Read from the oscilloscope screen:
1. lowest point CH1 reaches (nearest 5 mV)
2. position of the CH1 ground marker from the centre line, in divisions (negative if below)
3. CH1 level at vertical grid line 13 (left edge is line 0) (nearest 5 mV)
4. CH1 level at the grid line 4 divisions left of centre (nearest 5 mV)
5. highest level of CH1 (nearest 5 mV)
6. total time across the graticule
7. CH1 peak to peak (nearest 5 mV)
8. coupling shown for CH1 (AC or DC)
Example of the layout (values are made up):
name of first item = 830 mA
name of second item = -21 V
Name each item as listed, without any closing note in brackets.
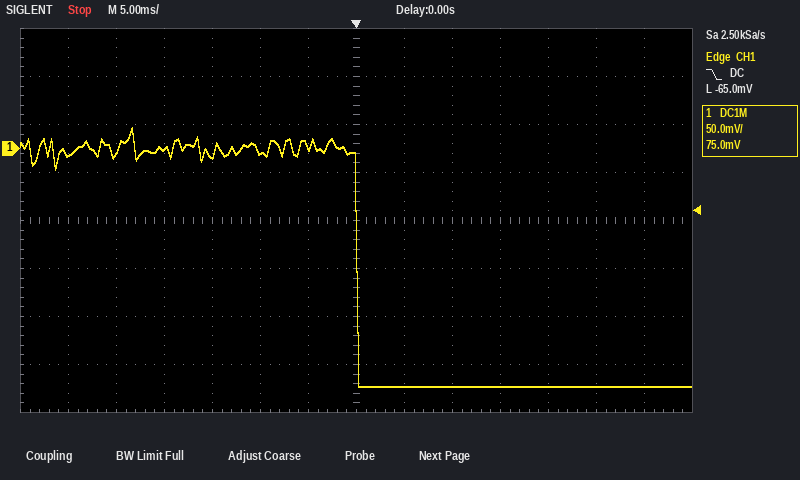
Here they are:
lowest point CH1 reaches = -250 mV
position of the CH1 ground marker from the centre line, in divisions = +1.5 div
CH1 level at vertical grid line 13 (left edge is line 0) = -250 mV
CH1 level at the grid line 4 divisions left of centre = 0 mV
highest level of CH1 = 20 mV
total time across the graticule = 70 ms
CH1 peak to peak = 270 mV
coupling shown for CH1 = DC
